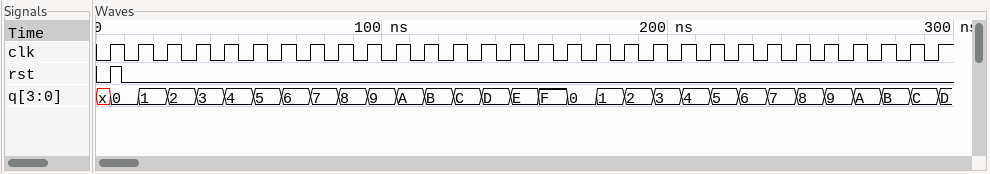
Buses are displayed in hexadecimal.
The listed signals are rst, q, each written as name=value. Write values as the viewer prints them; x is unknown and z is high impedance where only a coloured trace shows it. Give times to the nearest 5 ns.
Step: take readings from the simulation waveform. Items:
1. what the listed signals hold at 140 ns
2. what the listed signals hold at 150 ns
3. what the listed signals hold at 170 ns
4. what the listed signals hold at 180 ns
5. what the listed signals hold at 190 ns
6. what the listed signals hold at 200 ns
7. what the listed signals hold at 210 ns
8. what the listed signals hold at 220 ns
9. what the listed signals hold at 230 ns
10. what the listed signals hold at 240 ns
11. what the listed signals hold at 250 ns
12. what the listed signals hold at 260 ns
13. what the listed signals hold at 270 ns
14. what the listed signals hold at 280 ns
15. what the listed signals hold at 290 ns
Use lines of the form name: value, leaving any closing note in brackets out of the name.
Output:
what the listed signals hold at 140 ns: rst=0, q=D
what the listed signals hold at 150 ns: rst=0, q=E
what the listed signals hold at 170 ns: rst=0, q=0
what the listed signals hold at 180 ns: rst=0, q=1
what the listed signals hold at 190 ns: rst=0, q=2
what the listed signals hold at 200 ns: rst=0, q=3
what the listed signals hold at 210 ns: rst=0, q=4
what the listed signals hold at 220 ns: rst=0, q=5
what the listed signals hold at 230 ns: rst=0, q=6
what the listed signals hold at 240 ns: rst=0, q=7
what the listed signals hold at 250 ns: rst=0, q=8
what the listed signals hold at 260 ns: rst=0, q=9
what the listed signals hold at 270 ns: rst=0, q=A
what the listed signals hold at 280 ns: rst=0, q=B
what the listed signals hold at 290 ns: rst=0, q=C
